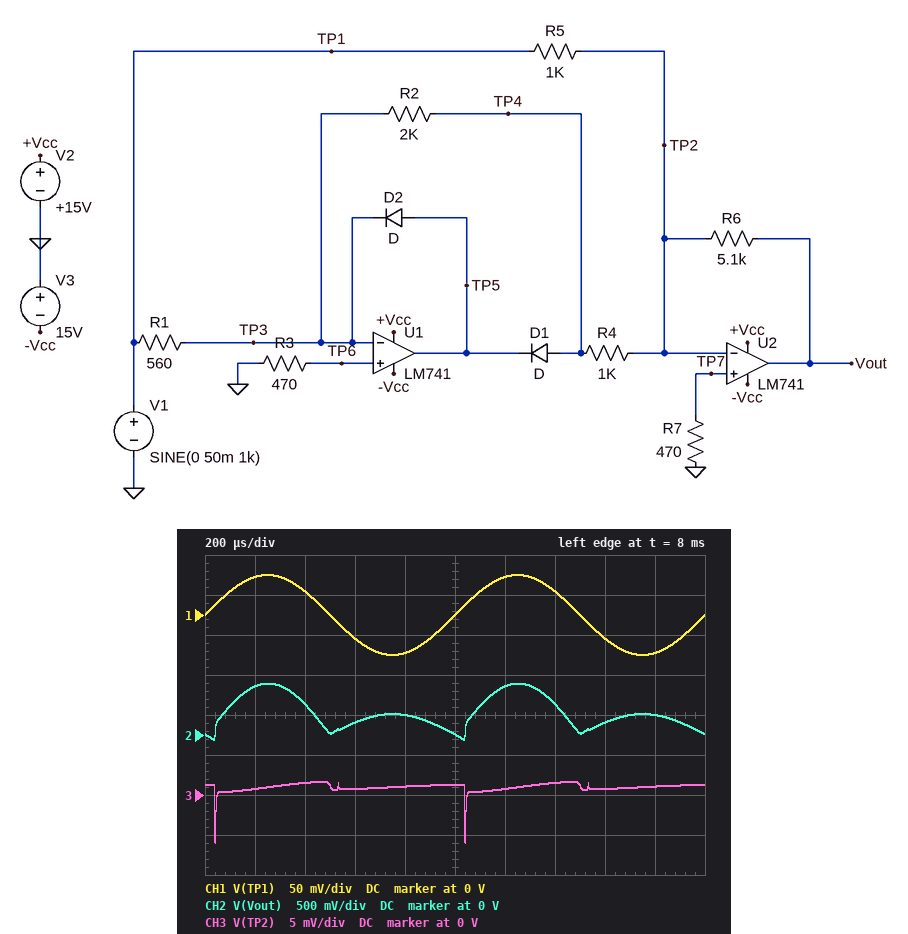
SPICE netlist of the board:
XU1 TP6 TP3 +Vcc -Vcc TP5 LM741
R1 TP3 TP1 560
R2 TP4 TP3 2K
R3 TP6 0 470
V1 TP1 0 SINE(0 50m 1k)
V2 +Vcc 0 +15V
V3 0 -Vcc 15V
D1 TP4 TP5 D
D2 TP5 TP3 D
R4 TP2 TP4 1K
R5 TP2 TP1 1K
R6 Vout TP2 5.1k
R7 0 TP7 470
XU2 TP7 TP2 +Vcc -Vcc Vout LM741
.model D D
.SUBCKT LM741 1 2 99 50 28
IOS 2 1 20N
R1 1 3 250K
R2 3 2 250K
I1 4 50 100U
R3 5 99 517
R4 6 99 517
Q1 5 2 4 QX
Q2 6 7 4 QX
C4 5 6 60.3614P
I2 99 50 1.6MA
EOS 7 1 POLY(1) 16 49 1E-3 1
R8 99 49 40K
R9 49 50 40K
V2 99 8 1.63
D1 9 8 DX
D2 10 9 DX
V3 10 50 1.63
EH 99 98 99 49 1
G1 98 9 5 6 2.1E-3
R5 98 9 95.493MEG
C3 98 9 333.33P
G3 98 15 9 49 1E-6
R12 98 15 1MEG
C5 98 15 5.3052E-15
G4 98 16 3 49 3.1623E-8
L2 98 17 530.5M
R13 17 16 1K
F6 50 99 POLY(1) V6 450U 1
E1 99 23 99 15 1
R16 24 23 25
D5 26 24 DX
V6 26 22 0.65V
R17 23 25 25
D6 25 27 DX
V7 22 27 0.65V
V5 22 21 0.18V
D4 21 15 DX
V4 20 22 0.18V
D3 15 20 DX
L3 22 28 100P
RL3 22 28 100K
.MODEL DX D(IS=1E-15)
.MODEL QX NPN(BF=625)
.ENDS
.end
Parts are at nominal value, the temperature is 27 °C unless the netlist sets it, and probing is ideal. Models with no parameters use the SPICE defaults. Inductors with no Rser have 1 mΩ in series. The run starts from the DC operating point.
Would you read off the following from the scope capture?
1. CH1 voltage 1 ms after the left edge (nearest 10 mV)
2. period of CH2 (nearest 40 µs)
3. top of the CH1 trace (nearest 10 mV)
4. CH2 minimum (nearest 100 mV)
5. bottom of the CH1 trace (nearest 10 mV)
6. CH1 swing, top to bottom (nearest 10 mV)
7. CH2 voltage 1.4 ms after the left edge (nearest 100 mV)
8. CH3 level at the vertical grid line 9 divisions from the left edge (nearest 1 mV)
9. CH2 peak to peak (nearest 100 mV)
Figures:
0 V
1.00 ms
50 mV
-100 mV
-50 mV
100 mV
400 mV
1 mV
700 mV
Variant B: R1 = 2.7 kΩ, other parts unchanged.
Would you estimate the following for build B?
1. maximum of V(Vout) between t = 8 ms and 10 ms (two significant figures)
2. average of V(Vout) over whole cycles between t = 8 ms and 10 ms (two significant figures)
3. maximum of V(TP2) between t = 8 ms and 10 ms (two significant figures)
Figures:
260 mV
63 mV
1.3 mV
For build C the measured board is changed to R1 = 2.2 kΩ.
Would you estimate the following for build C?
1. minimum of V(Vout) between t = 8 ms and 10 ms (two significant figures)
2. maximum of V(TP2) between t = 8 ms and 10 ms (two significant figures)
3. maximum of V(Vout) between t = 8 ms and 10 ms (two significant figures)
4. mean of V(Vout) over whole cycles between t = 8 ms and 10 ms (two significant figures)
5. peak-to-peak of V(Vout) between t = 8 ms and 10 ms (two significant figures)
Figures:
-71 mV
1.3 mV
260 mV
76 mV
330 mV
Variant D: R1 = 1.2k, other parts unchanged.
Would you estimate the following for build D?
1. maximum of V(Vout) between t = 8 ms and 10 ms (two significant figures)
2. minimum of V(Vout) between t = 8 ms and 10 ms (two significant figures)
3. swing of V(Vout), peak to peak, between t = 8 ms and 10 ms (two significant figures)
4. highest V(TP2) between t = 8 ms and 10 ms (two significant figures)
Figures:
260 mV
-67 mV
330 mV
1.4 mV
